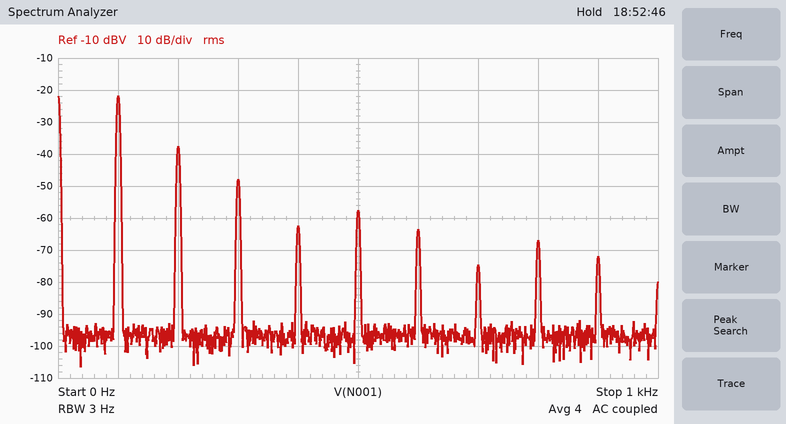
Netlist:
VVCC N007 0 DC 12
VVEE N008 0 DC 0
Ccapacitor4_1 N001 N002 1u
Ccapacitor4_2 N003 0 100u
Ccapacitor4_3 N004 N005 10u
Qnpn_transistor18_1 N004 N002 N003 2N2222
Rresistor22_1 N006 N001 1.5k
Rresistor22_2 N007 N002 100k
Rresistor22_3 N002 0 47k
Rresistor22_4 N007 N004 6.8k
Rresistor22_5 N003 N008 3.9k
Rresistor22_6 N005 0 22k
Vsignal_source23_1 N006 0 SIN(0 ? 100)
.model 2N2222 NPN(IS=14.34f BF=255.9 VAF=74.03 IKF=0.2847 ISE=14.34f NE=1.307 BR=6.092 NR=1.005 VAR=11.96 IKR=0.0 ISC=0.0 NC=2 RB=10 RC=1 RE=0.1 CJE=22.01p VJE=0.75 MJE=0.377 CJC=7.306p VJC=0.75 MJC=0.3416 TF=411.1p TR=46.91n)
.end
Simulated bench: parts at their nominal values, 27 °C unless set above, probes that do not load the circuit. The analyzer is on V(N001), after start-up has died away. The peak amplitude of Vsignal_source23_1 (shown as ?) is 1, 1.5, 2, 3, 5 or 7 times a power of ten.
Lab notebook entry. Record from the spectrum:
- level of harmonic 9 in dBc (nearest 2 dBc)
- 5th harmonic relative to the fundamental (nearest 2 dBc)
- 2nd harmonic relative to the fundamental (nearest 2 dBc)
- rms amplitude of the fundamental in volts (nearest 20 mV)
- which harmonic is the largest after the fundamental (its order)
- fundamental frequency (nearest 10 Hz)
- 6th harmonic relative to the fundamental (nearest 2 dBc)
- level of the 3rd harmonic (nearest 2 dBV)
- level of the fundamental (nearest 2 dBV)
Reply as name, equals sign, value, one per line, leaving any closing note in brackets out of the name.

level of harmonic 9 in dBc = -50 dBc
5th harmonic relative to the fundamental = -36 dBc
2nd harmonic relative to the fundamental = -16 dBc
rms amplitude of the fundamental in volts = 80 mV
which harmonic is the largest after the fundamental = 2
fundamental frequency = 100 Hz
6th harmonic relative to the fundamental = -42 dBc
level of the 3rd harmonic = -48 dBV
level of the fundamental = -22 dBV
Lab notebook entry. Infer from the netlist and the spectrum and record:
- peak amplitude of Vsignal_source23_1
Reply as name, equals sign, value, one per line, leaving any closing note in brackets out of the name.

peak amplitude of Vsignal_source23_1 = 150 mV
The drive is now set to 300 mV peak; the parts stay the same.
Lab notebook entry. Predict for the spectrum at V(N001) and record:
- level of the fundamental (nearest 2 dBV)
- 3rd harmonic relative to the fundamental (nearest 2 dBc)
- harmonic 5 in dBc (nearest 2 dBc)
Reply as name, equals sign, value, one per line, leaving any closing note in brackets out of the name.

level of the fundamental = -16 dBV
3rd harmonic relative to the fundamental = -24 dBc
harmonic 5 in dBc = -34 dBc
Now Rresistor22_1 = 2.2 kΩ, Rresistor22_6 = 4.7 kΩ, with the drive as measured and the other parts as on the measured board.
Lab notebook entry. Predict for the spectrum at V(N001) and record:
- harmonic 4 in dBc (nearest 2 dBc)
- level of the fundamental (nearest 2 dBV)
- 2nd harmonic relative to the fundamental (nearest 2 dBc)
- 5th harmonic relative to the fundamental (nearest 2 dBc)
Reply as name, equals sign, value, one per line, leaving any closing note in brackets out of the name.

harmonic 4 in dBc = -38 dBc
level of the fundamental = -22 dBV
2nd harmonic relative to the fundamental = -18 dBc
5th harmonic relative to the fundamental = -60 dBc
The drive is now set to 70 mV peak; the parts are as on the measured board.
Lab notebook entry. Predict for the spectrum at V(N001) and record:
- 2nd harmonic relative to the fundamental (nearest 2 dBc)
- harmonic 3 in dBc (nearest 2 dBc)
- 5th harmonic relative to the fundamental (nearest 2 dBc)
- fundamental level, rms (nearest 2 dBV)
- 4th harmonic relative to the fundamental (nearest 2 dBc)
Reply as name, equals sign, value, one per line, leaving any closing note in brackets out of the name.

2nd harmonic relative to the fundamental = -18 dBc
harmonic 3 in dBc = -28 dBc
5th harmonic relative to the fundamental = -52 dBc
fundamental level, rms = -28 dBV
4th harmonic relative to the fundamental = -40 dBc
